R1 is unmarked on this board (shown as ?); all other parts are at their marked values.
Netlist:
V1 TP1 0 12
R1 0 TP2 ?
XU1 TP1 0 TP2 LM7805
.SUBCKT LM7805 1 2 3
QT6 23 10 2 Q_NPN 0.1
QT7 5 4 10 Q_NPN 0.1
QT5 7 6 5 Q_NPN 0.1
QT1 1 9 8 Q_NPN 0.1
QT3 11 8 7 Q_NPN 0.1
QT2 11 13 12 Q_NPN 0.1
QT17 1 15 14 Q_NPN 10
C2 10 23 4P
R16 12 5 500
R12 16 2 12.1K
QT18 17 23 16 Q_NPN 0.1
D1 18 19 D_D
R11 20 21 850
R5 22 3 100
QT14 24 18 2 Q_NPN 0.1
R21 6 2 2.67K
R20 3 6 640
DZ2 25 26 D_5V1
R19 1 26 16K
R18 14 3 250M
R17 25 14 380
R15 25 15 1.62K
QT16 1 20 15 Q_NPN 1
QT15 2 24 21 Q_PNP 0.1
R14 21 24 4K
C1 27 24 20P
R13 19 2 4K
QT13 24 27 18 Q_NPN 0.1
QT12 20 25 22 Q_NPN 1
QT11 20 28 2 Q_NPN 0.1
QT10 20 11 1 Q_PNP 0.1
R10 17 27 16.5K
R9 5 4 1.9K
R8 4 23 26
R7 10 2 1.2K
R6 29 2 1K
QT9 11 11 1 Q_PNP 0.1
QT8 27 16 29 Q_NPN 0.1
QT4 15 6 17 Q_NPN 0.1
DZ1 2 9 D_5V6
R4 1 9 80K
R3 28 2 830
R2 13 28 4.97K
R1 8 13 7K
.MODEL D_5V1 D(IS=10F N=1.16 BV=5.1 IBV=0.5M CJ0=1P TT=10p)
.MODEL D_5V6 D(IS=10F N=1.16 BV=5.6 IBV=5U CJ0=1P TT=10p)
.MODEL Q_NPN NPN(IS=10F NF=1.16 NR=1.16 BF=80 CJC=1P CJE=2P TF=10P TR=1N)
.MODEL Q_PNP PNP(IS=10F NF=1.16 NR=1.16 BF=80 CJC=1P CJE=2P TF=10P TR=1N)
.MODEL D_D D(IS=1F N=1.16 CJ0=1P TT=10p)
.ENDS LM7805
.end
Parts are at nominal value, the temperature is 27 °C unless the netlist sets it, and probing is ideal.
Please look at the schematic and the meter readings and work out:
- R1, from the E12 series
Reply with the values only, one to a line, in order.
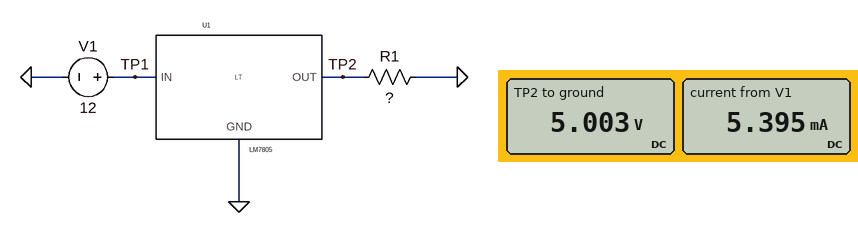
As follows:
15 kΩ
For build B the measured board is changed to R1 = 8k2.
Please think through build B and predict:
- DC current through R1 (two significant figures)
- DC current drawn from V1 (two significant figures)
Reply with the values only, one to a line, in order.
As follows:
610 µA
5.7 mA
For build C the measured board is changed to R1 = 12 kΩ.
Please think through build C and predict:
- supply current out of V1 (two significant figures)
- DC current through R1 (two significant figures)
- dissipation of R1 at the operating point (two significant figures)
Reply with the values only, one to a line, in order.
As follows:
5.5 mA
420 µA
2.1 mW
